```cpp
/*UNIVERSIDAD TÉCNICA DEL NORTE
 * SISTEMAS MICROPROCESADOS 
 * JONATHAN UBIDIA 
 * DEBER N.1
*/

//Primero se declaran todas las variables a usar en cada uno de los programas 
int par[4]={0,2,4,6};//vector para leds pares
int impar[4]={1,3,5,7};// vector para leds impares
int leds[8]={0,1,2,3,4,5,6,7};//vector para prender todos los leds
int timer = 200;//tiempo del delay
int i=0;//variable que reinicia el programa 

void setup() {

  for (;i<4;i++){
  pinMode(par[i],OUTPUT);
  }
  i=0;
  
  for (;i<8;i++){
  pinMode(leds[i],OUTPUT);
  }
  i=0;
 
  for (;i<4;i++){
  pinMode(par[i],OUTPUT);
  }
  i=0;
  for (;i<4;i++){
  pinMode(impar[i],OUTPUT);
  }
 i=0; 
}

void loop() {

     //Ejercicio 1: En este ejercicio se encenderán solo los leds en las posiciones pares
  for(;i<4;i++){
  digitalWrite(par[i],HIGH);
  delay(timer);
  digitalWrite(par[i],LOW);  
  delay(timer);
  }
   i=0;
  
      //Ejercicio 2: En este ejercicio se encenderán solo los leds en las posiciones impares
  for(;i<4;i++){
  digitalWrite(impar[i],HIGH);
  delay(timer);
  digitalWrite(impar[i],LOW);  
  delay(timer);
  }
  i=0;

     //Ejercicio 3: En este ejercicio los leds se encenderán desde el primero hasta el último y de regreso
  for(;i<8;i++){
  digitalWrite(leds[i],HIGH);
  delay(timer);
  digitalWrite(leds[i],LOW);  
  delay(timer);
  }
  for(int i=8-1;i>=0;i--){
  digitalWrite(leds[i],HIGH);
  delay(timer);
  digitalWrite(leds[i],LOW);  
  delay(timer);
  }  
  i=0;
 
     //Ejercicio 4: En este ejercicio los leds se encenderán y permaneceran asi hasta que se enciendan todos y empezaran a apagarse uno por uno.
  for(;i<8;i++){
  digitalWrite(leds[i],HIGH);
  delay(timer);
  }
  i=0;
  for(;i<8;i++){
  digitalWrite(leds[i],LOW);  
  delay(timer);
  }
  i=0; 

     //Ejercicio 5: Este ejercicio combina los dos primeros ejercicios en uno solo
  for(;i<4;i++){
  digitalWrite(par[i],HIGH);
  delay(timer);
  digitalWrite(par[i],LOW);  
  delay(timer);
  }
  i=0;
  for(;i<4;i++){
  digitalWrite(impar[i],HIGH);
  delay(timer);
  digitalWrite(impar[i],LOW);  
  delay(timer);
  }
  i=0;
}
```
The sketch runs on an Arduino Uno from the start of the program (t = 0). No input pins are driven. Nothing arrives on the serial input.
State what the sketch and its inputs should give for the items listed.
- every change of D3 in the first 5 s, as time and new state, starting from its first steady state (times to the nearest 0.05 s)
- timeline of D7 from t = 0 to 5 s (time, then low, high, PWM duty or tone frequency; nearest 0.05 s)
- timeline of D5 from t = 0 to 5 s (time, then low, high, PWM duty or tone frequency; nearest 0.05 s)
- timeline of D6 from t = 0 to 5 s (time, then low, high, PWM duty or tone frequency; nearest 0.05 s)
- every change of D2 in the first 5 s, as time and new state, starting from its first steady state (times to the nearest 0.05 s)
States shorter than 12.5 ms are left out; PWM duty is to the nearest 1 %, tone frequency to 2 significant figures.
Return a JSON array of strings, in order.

["0 s low; 2 s high; 2.2 s low; 4.4 s high; 4.6 s low", "0 s low; 2.8 s high; 3 s low", "0 s low; 2.4 s high; 2.6 s low", "0 s low; 1.2 s high; 1.4 s low", "0 s low; 0.4 s high; 0.6 s low; 4 s high; 4.2 s low"]
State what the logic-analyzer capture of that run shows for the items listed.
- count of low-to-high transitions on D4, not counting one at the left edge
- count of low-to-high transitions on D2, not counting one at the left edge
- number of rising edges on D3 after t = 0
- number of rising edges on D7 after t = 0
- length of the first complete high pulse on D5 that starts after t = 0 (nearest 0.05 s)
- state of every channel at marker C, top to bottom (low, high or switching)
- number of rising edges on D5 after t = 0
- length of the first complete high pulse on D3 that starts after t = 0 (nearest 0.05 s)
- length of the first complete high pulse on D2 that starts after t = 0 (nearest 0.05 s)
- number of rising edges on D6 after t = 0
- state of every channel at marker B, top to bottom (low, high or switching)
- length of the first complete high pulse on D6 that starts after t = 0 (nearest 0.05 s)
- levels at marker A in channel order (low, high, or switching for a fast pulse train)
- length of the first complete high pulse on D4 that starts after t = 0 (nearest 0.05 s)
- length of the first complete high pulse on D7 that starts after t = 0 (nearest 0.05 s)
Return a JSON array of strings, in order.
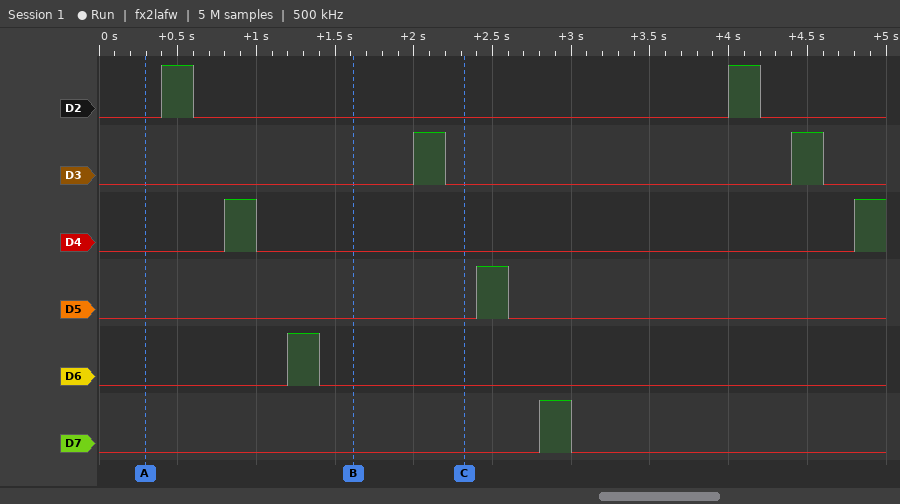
["2", "2", "2", "1", "0.20 s", "D2 low, D3 low, D4 low, D5 low, D6 low, D7 low", "1", "0.20 s", "0.20 s", "1", "D2 low, D3 low, D4 low, D5 low, D6 low, D7 low", "0.20 s", "D2 low, D3 low, D4 low, D5 low, D6 low, D7 low", "0.20 s", "0.20 s"]
